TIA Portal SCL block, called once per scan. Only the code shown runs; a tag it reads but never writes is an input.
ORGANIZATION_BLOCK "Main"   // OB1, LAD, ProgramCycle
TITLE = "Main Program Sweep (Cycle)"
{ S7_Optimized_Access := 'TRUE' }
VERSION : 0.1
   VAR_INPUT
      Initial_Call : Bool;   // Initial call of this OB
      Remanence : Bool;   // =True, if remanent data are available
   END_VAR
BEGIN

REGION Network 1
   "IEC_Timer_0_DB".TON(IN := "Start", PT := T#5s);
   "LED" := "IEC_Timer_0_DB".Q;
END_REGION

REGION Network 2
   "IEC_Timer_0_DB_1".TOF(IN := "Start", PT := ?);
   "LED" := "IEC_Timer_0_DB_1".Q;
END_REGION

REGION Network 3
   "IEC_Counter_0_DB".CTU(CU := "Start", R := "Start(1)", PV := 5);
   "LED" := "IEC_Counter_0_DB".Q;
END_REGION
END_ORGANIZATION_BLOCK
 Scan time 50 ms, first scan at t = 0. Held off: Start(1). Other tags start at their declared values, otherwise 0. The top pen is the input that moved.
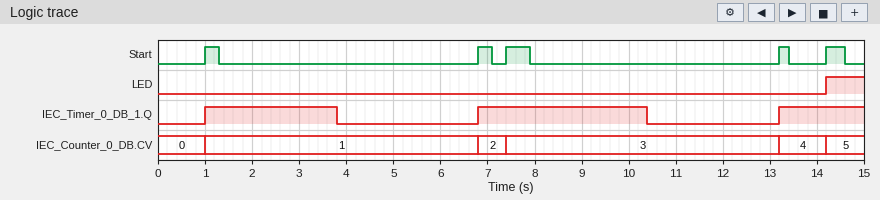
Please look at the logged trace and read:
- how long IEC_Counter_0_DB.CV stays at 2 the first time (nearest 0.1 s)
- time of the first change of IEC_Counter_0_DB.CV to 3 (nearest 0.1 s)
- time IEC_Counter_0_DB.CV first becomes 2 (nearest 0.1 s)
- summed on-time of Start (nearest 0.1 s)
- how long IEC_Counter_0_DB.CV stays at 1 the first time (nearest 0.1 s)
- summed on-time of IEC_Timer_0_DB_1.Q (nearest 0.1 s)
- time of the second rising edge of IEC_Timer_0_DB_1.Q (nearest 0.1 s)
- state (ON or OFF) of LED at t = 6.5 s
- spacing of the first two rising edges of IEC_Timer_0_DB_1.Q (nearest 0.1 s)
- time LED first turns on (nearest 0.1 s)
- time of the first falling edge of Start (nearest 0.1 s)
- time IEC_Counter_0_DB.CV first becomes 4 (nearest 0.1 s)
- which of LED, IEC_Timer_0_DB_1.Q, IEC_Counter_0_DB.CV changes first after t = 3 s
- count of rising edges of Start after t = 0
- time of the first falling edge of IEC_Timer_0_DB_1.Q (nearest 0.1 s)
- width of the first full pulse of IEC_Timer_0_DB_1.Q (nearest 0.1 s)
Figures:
0.6 s
7.4 s
6.8 s
1.7 s
5.8 s
8.2 s
6.8 s
OFF
5.8 s
14.2 s
1.3 s
13.2 s
IEC_Timer_0_DB_1.Q
5
3.8 s
2.8 s
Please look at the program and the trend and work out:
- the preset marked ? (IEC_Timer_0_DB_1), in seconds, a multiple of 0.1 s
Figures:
2.5 s
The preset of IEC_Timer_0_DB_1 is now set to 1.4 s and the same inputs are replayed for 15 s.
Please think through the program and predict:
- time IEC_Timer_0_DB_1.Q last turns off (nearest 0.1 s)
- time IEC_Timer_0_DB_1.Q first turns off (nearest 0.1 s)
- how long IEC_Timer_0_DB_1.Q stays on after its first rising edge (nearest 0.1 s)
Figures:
9.3 s
2.7 s
1.7 s
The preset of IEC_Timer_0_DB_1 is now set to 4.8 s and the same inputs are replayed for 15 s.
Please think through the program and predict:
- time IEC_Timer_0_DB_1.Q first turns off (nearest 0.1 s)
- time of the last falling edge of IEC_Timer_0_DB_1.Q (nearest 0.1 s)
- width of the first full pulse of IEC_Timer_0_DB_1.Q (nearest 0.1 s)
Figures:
6.1 s
12.7 s
5.1 s
